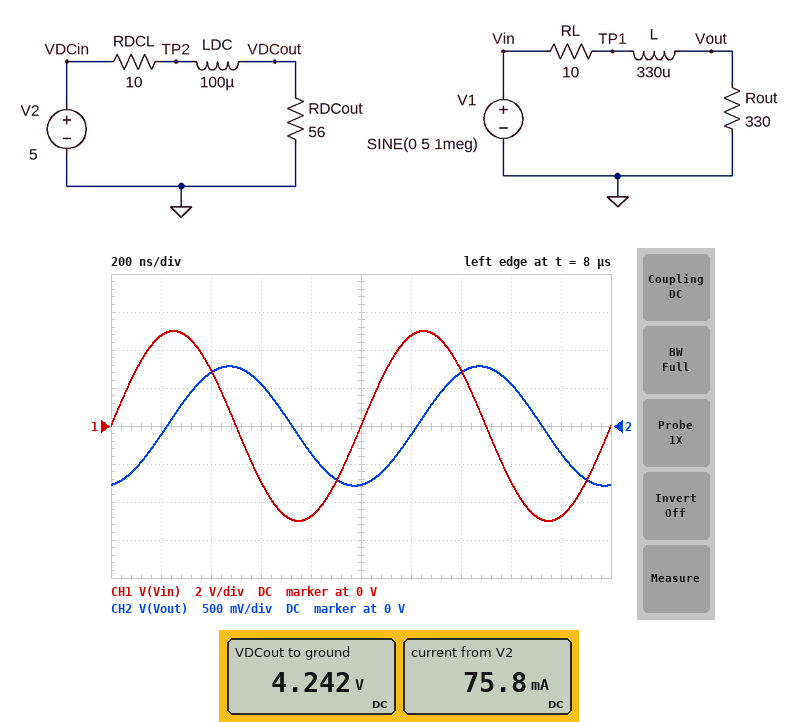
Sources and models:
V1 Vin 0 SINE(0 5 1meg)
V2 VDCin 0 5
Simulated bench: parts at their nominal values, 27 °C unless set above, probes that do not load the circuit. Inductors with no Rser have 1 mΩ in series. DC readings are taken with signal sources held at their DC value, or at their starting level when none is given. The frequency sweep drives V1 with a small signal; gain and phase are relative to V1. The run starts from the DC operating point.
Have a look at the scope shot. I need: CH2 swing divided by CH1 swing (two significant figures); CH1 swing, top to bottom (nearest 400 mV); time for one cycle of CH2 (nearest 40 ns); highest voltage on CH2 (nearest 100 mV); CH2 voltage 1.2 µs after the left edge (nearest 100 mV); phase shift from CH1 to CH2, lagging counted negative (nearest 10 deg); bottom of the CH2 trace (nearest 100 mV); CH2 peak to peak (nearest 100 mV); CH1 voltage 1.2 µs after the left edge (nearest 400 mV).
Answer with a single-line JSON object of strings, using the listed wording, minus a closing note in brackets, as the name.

{"CH2 swing divided by CH1 swing": "0.16", "CH1 swing, top to bottom": "10.0 V", "time for one cycle of CH2": "1.00 µs", "highest voltage on CH2": "800 mV", "CH2 voltage 1.2 µs after the left edge": "-100 mV", "phase shift from CH1 to CH2, lagging counted negative": "-80 deg", "bottom of the CH2 trace": "-800 mV", "CH2 peak to peak": "1.6 V", "CH1 voltage 1.2 µs after the left edge": "4.8 V"}
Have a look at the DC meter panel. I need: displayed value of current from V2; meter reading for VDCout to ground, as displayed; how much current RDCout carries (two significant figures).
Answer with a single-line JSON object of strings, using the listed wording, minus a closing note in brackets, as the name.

{"displayed value of current from V2": "75.8 mA", "meter reading for VDCout to ground, as displayed": "4.242 V", "how much current RDCout carries": "76 mA"}
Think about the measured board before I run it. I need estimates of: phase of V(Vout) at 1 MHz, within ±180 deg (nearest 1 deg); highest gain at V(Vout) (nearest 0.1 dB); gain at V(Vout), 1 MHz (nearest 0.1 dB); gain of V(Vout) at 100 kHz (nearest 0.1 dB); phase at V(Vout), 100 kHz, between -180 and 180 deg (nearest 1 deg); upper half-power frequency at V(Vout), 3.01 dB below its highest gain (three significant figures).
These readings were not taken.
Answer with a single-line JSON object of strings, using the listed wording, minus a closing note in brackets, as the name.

{"phase of V(Vout) at 1 MHz, within ±180 deg": "-81 deg", "highest gain at V(Vout)": "-0.3 dB", "gain at V(Vout), 1 MHz": "-16.1 dB", "gain of V(Vout) at 100 kHz": "-1.6 dB", "phase at V(Vout), 100 kHz, between -180 and 180 deg": "-31 deg", "upper half-power frequency at V(Vout), 3.01 dB below its highest gain": "164 kHz"}
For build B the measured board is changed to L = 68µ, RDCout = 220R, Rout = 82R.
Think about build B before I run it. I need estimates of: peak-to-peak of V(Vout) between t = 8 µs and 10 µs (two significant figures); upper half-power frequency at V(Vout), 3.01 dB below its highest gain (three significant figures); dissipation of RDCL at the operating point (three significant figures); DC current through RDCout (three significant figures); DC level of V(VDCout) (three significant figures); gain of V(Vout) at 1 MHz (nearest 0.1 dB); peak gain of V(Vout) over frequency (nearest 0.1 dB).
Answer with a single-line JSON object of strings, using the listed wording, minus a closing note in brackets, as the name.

{"peak-to-peak of V(Vout) between t = 8 µs and 10 µs": "1.9 V", "upper half-power frequency at V(Vout), 3.01 dB below its highest gain": "215 kHz", "dissipation of RDCL at the operating point": "4.73 mW", "DC current through RDCout": "21.7 mA", "DC level of V(VDCout)": "4.78 V", "gain of V(Vout) at 1 MHz": "-14.5 dB", "peak gain of V(Vout) over frequency": "-1.0 dB"}
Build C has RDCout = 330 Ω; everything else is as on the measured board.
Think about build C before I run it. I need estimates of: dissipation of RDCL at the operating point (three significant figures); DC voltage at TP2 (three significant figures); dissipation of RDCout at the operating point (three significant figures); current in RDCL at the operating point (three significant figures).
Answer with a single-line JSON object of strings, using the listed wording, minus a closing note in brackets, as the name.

{"dissipation of RDCL at the operating point": "2.16 mW", "DC voltage at TP2": "4.85 V", "dissipation of RDCout at the operating point": "71.4 mW", "current in RDCL at the operating point": "14.7 mA"}
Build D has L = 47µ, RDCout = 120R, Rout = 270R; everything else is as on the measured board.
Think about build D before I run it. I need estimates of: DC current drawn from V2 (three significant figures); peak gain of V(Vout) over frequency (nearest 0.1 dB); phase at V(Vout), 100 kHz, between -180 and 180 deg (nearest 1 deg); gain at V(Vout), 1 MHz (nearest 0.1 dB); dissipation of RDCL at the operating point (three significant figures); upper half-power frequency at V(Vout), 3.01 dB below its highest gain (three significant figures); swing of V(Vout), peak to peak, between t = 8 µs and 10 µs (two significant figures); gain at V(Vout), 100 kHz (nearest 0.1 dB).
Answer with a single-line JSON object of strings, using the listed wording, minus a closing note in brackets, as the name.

{"DC current drawn from V2": "38.5 mA", "peak gain of V(Vout) over frequency": "-0.3 dB", "phase at V(Vout), 100 kHz, between -180 and 180 deg": "-6 deg", "gain at V(Vout), 1 MHz": "-3.6 dB", "dissipation of RDCL at the operating point": "14.8 mW", "upper half-power frequency at V(Vout), 3.01 dB below its highest gain": "948 kHz", "swing of V(Vout), peak to peak, between t = 8 µs and 10 µs": "6.6 V", "gain at V(Vout), 100 kHz": "-0.4 dB"}
